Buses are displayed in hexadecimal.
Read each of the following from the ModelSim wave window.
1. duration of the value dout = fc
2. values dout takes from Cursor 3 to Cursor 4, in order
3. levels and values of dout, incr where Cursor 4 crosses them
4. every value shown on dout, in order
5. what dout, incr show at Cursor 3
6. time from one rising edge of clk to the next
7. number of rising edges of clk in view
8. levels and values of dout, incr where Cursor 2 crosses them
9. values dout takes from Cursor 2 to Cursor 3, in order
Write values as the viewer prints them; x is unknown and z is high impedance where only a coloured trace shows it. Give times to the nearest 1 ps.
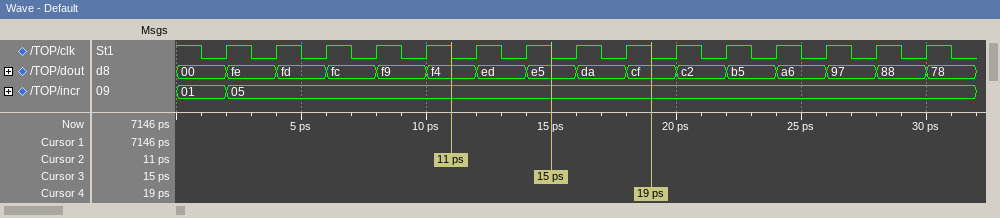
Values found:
2 ps
e5, da, cf
dout=cf, incr=05
00, fe, fd, fc, f9, f4, ed, e5, da, cf, c2, b5, a6, 97, 88, 78
dout=e5, incr=05
2 ps
15
dout=f4, incr=05
f4, ed, e5
